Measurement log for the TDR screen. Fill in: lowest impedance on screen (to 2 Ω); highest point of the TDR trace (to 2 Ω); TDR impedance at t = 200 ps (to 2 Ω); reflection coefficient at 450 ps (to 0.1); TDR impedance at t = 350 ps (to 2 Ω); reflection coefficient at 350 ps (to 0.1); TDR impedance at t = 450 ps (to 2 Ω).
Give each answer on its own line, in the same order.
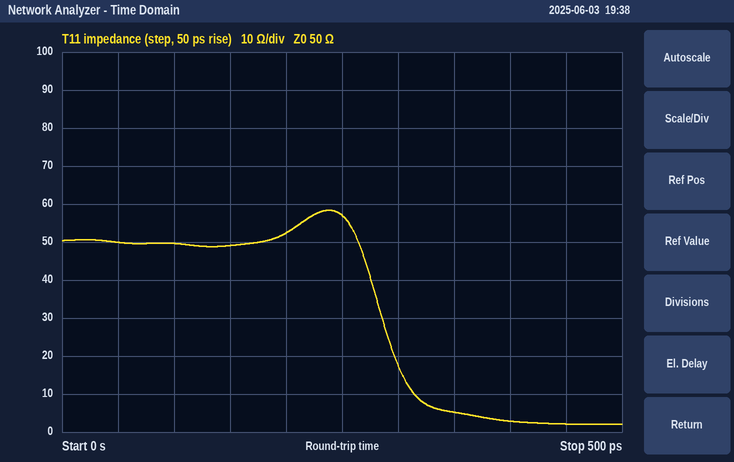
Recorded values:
2 Ω
58 Ω
52 Ω
-0.9
6 Ω
-0.8
2 Ω
